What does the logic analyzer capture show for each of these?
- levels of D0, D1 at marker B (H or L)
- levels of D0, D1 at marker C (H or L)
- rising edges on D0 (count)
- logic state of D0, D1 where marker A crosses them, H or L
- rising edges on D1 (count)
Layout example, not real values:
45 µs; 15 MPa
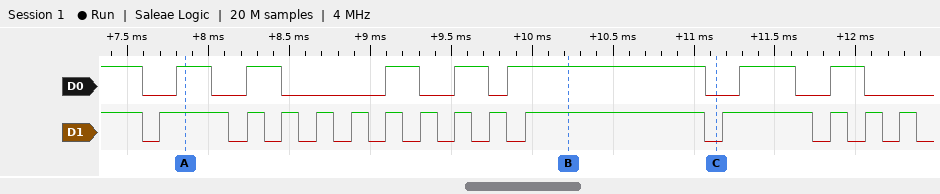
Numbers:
D0=H, D1=H; D0=L, D1=L; 7; D0=H, D1=H; 14
